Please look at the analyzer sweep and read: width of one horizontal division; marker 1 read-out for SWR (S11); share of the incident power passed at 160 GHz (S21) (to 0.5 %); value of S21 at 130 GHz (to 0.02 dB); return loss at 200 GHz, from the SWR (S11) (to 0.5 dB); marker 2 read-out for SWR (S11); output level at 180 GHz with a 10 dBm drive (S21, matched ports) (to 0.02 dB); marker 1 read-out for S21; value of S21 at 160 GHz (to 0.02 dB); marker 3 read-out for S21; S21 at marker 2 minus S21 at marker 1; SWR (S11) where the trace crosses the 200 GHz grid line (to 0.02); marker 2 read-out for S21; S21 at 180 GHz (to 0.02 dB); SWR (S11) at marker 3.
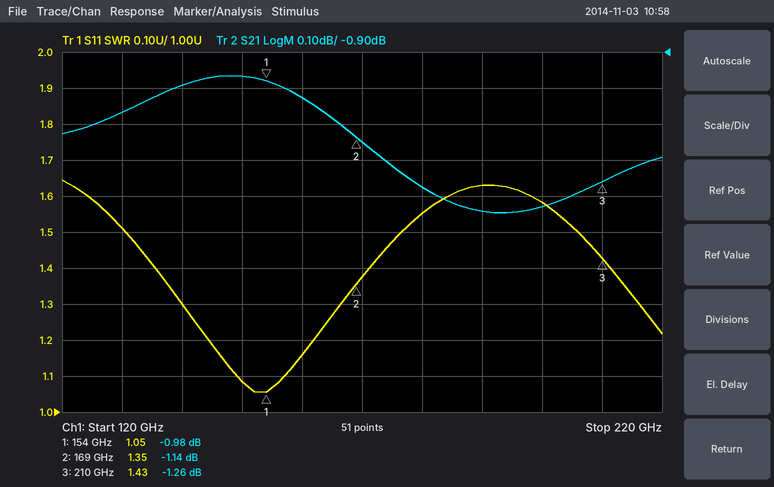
10 GHz
1.05
79.0 %
-1.06 dB
13.0 dB
1.35
8.72 dBm
-0.98 dB
-1.02 dB
-1.26 dB
-0.16 dB
1.58
-1.14 dB
-1.28 dB
1.43
